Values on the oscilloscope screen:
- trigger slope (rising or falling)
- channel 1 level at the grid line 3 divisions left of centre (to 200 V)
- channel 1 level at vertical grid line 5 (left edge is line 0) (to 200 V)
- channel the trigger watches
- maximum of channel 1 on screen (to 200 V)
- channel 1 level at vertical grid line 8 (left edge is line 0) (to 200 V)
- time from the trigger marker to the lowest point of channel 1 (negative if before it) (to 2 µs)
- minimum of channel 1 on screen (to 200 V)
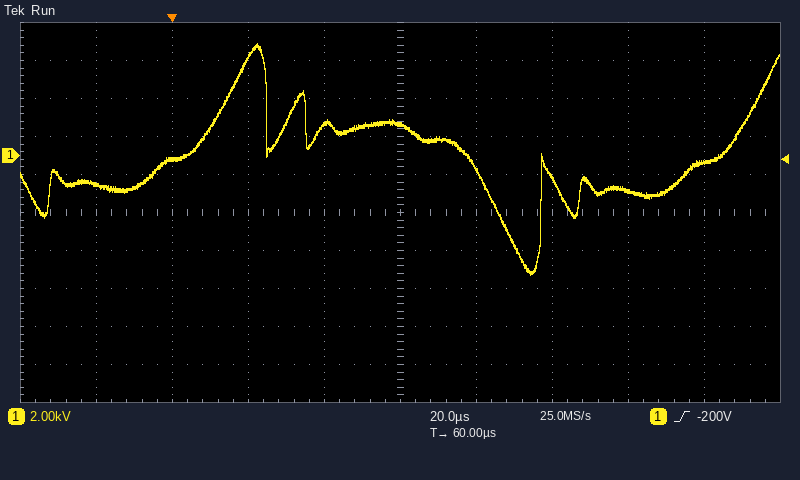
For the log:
rising
-200 V
1.6 kV
channel 1
5.8 kV
-1.8 kV
+94 µs
-6.2 kV
